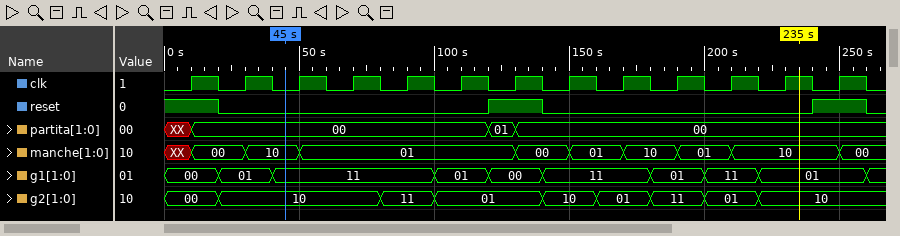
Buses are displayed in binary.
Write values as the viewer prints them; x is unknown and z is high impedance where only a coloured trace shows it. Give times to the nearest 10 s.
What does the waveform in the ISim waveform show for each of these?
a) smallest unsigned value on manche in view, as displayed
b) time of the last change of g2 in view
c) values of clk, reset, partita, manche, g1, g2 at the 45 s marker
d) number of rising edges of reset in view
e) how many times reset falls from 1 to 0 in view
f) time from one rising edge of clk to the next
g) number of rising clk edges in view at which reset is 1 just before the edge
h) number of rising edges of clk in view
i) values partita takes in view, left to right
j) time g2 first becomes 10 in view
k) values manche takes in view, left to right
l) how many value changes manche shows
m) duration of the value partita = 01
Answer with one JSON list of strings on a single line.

["00", "220 s", "clk=0, reset=0, partita=00, manche=10, g1=11, g2=10", "2", "3", "20 s", "3", "13", "XX, 00, 01, 00", "20 s", "XX, 00, 10, 01, 00, 01, 10, 01, 10, 00", "9", "10 s"]
